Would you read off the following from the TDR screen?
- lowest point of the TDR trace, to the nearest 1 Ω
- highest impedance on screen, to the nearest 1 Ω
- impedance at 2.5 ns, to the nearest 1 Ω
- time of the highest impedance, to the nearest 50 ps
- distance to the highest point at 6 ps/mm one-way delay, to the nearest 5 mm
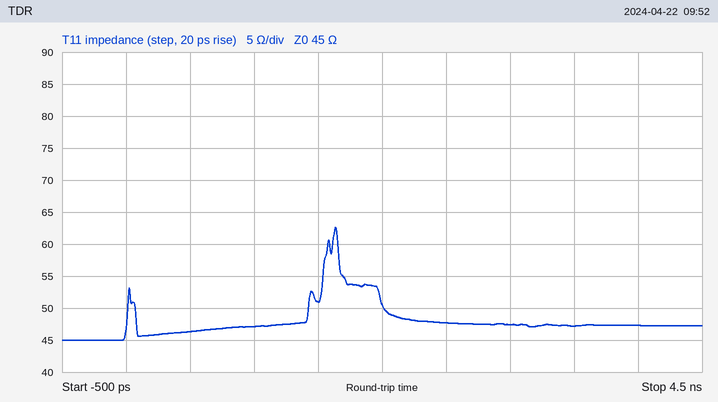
45 Ω
63 Ω
48 Ω
1.65 ns
135 mm
